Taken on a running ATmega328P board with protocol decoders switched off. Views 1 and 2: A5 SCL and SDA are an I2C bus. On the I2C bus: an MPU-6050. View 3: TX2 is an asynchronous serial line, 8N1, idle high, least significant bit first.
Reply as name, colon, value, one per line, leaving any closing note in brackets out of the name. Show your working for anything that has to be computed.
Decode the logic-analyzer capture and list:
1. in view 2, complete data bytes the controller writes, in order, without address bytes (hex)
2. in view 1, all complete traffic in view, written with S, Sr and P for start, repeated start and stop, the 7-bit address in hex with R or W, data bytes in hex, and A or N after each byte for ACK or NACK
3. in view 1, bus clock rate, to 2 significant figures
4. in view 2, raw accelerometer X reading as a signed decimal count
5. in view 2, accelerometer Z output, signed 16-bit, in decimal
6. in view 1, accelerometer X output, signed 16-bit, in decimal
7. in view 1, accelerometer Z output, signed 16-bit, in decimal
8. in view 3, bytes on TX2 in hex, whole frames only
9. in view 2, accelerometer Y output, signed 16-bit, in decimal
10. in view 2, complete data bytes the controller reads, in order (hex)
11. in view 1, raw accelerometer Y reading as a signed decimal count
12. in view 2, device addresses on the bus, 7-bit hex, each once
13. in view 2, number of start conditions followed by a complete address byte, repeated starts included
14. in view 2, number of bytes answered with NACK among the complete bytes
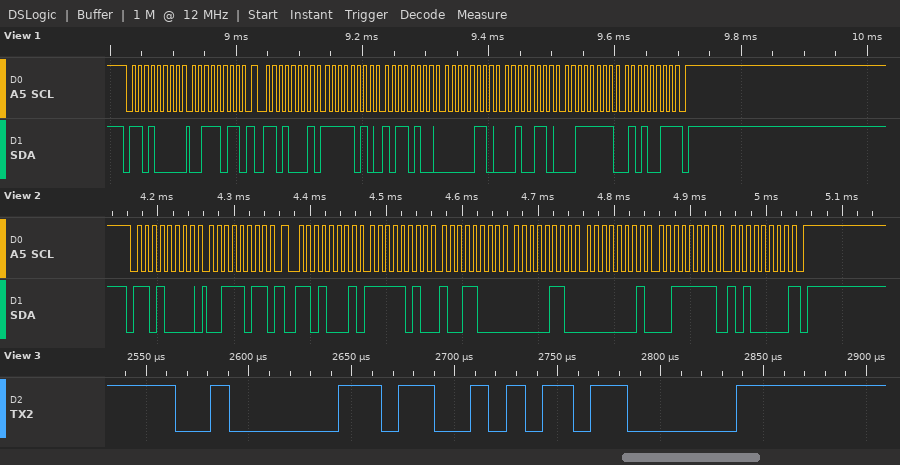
in view 2, complete data bytes the controller writes, in order, without address bytes: 3B
in view 1, all complete traffic in view, written with S, Sr and P for start, repeated start and stop, the 7-bit address in hex with R or W, data bytes in hex, and A or N after each byte for ACK or NACK: S 68W A 3B A Sr 68R A FA A B4 A 06 A 26 A 3F A 53 N P
in view 1, bus clock rate, to 2 significant figures: 100 kHz
in view 2, raw accelerometer X reading as a signed decimal count: 0xFA98 = -1384
in view 2, accelerometer Z output, signed 16-bit, in decimal: 0x3FA0 = 16288
in view 1, accelerometer X output, signed 16-bit, in decimal: 0xFAB4 = -1356
in view 1, accelerometer Z output, signed 16-bit, in decimal: 0x3F53 = 16211
in view 3, bytes on TX2 in hex, whole frames only: 02 53 03
in view 2, accelerometer Y output, signed 16-bit, in decimal: 0x0601 = 1537
in view 2, complete data bytes the controller reads, in order: FA 98 06 01 3F A0
in view 1, raw accelerometer Y reading as a signed decimal count: 0x0626 = 1574
in view 2, device addresses on the bus, 7-bit hex, each once: 0x68
in view 2, number of start conditions followed by a complete address byte, repeated starts included: 2
in view 2, number of bytes answered with NACK among the complete bytes: 1
